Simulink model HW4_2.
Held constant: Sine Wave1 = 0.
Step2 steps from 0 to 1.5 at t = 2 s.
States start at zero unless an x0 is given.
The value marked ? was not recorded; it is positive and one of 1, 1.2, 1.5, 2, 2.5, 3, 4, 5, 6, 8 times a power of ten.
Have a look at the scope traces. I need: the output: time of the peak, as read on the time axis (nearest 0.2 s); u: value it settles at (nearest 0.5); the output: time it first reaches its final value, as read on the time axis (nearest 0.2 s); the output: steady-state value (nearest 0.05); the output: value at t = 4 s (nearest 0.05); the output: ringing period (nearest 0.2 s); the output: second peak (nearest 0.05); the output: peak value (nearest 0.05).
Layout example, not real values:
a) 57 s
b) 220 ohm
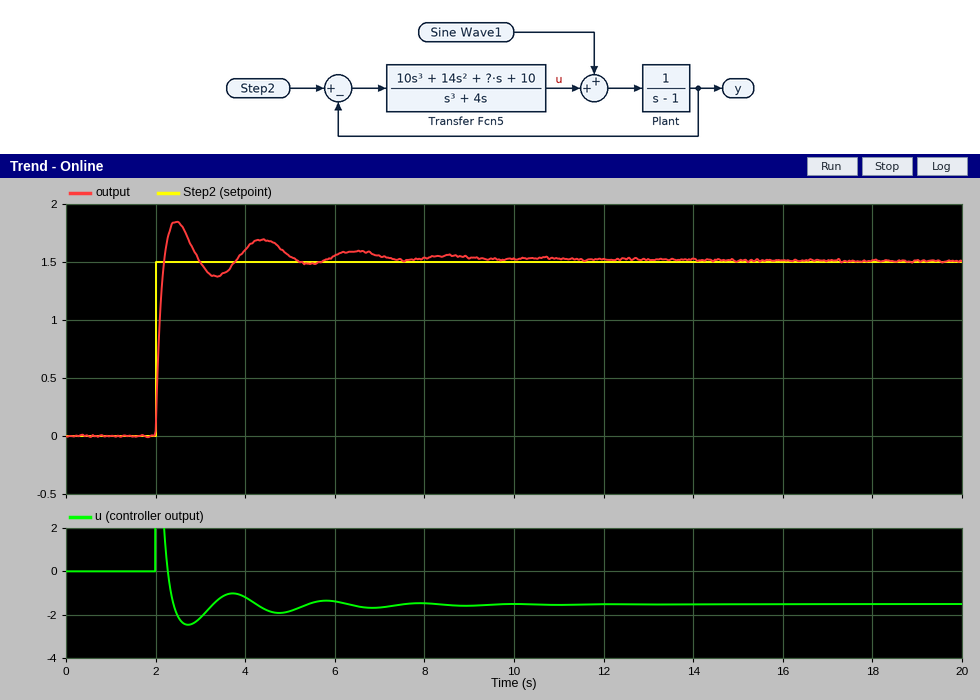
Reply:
a) 2.4 s
b) -1.5
c) 2.2 s
d) 1.50
e) 1.60
f) 2.0 s
g) 1.70
h) 1.85
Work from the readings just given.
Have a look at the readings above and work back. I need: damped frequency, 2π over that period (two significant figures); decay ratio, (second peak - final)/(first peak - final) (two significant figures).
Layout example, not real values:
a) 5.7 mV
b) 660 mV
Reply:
a) 3.1 rad/s
b) 0.57
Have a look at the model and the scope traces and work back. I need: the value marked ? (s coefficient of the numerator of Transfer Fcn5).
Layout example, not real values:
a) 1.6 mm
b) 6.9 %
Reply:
a) 80
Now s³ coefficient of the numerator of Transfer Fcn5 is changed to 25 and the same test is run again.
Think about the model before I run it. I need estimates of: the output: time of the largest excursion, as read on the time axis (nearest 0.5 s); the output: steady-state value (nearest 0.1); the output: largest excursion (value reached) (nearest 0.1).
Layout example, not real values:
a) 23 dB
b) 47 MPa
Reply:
a) 4.5 s
b) 1.5
c) 1.6
